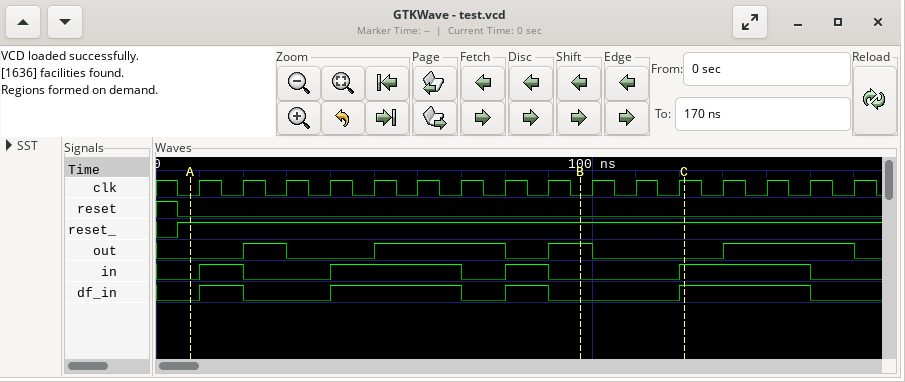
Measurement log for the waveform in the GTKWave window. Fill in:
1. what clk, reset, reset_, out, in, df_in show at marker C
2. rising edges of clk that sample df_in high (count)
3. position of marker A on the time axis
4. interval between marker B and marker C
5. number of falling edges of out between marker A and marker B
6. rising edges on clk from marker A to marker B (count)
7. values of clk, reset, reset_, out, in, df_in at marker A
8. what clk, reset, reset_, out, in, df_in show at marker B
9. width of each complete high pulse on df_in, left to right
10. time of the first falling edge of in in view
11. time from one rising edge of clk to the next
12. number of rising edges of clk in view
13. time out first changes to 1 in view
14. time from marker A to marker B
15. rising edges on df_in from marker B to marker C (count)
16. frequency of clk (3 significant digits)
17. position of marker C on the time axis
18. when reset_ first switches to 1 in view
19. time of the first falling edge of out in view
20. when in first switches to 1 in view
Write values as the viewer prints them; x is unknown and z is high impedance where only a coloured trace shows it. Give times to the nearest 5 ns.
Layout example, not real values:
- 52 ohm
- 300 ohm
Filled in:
- clk=1, reset=0, reset_=1, out=0, in=1, df_in=1
- 8
- 10 ns
- 25 ns
- 2
- 9
- clk=0, reset=0, reset_=1, out=0, in=0, df_in=0
- clk=0, reset=0, reset_=1, out=1, in=0, df_in=0
- 10 ns, 30 ns, 10 ns, 30 ns
- 20 ns
- 10 ns
- 16
- 20 ns
- 90 ns
- 1
- 100 MHz
- 120 ns
- 5 ns
- 30 ns
- 10 ns
